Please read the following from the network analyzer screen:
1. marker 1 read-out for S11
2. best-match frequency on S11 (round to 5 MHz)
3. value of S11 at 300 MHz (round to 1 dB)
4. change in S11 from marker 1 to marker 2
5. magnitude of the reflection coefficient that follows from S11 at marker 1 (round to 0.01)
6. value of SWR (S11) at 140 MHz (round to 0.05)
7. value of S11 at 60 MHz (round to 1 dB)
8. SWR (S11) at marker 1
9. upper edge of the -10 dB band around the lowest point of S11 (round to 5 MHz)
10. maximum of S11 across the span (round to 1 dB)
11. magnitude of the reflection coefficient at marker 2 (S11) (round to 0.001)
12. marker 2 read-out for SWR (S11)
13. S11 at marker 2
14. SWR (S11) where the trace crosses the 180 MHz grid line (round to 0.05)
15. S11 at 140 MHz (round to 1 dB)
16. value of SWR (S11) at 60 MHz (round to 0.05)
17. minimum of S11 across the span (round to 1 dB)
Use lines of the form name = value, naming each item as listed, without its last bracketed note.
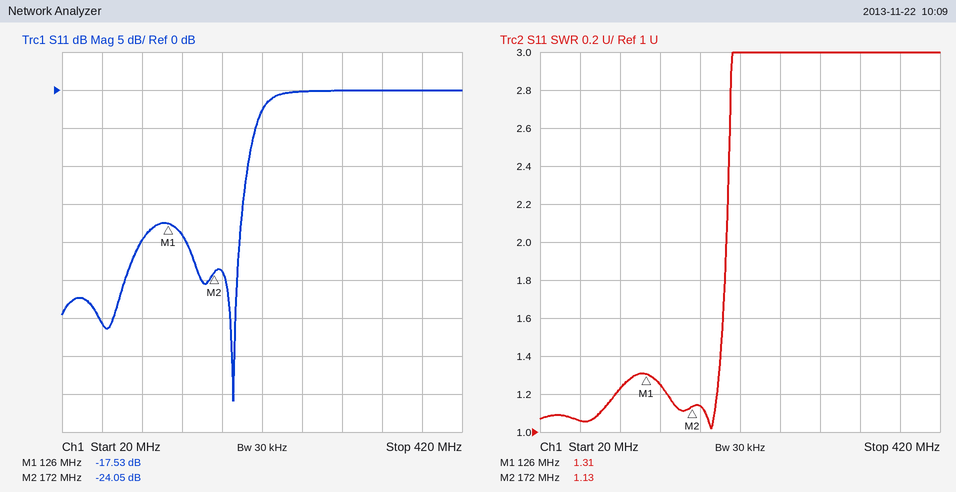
marker 1 read-out for S11 = -17.53 dB
best-match frequency on S11 = 190 MHz
value of S11 at 300 MHz = 0 dB
change in S11 from marker 1 to marker 2 = -6.52 dB
magnitude of the reflection coefficient that follows from S11 at marker 1 = 0.13
value of SWR (S11) at 140 MHz = 1.25
value of S11 at 60 MHz = -31 dB
SWR (S11) at marker 1 = 1.31
upper edge of the -10 dB band around the lowest point of S11 = 205 MHz
maximum of S11 across the span = 0 dB
magnitude of the reflection coefficient at marker 2 (S11) = 0.063
marker 2 read-out for SWR = 1.13
S11 at marker 2 = -24.05 dB
SWR (S11) where the trace crosses the 180 MHz grid line = 1.15
S11 at 140 MHz = -19 dB
value of SWR (S11) at 60 MHz = 1.05
minimum of S11 across the span = -41 dB
